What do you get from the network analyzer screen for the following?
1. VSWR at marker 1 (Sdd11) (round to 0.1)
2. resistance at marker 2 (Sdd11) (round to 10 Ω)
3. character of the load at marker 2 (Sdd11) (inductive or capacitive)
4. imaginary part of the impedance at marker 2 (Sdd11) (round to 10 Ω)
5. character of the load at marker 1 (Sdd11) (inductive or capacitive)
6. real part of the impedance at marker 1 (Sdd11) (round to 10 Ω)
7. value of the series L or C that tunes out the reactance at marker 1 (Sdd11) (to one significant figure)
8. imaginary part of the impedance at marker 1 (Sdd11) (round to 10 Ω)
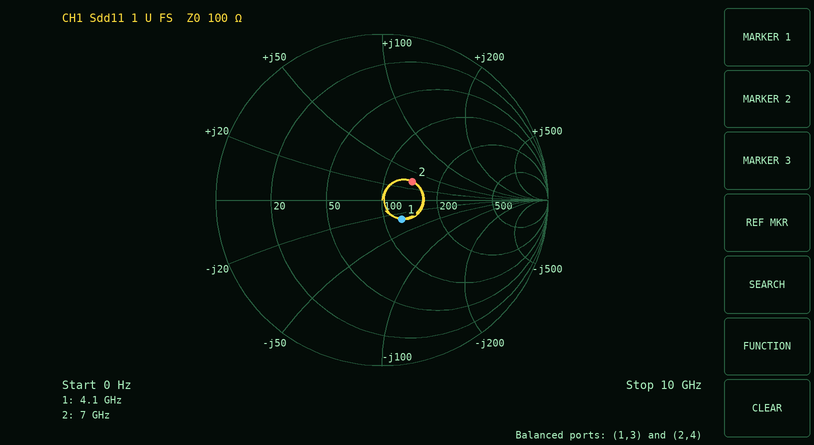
1.4
140 Ω
inductive
+30 Ω
capacitive
120 Ω
1 nH
-30 Ω
